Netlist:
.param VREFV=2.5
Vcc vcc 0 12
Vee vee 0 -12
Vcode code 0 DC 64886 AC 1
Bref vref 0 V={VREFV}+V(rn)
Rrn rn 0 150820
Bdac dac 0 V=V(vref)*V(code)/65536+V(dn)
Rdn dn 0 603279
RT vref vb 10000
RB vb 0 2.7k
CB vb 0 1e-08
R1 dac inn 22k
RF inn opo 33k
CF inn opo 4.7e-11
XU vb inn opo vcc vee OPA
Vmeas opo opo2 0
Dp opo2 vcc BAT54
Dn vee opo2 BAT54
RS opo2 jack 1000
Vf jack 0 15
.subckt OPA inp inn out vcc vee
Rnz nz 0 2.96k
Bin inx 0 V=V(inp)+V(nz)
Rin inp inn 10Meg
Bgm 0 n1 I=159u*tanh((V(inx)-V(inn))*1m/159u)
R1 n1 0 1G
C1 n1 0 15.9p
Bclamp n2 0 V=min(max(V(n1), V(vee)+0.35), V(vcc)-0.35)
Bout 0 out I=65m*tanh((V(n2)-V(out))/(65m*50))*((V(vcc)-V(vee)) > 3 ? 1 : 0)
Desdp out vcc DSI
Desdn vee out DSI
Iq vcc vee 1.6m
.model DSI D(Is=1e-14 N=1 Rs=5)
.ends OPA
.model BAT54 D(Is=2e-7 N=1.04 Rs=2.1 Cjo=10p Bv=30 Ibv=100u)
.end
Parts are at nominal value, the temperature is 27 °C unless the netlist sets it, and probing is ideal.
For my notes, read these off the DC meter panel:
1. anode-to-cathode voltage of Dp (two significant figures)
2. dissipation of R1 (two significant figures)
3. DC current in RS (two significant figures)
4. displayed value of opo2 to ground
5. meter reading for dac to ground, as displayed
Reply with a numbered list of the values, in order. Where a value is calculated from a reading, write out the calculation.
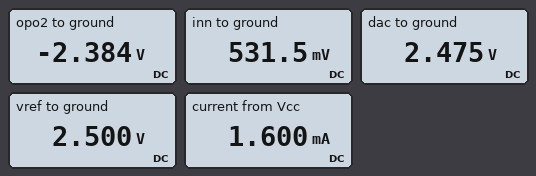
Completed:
1. -2.384 V - 12 V = -14 V
2. (2.475 V - 531.5 mV)^2 / 22 kΩ = 170 µW
3. (15 V - (-2.384 V)) / 1 kΩ = 17 mA
4. -2.384 V
5. 2.475 V
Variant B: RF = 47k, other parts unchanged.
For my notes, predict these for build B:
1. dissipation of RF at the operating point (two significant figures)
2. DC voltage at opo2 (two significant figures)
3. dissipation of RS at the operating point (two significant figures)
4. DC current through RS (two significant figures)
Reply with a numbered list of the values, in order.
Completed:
1. 370 µW
2. -3.6 V
3. 350 mW
4. 19 mA
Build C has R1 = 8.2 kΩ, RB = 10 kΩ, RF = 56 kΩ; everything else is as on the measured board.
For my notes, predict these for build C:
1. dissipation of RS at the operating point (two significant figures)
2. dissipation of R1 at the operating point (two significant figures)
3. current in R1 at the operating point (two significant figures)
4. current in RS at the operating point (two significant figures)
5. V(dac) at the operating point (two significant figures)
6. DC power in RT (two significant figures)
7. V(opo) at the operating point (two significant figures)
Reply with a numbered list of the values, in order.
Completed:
1. 490 mW
2. 180 µW
3. 150 µA
4. 22 mA
5. 2.5 V
6. 160 µW
7. -7.1 V
